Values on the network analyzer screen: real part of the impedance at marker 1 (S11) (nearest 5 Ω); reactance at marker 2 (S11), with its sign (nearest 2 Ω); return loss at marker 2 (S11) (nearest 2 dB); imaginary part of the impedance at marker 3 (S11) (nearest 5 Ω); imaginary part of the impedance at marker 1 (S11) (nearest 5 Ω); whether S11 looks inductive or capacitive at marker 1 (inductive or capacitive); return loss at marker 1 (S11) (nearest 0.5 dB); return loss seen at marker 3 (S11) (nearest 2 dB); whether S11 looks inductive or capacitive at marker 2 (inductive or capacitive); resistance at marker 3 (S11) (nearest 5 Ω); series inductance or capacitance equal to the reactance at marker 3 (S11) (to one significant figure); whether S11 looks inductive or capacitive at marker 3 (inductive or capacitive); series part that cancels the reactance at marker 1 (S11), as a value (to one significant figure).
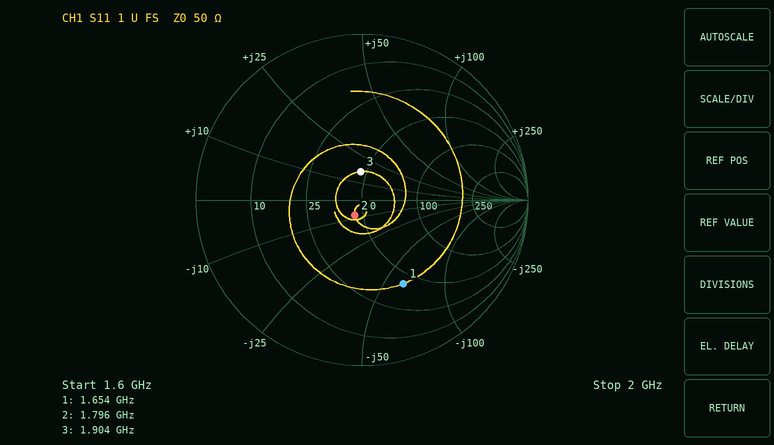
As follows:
40 Ω
-8 Ω
20 dB
+15 Ω
-60 Ω
capacitive
5.0 dB
16 dB
capacitive
45 Ω
1 nH
inductive
6 nH
